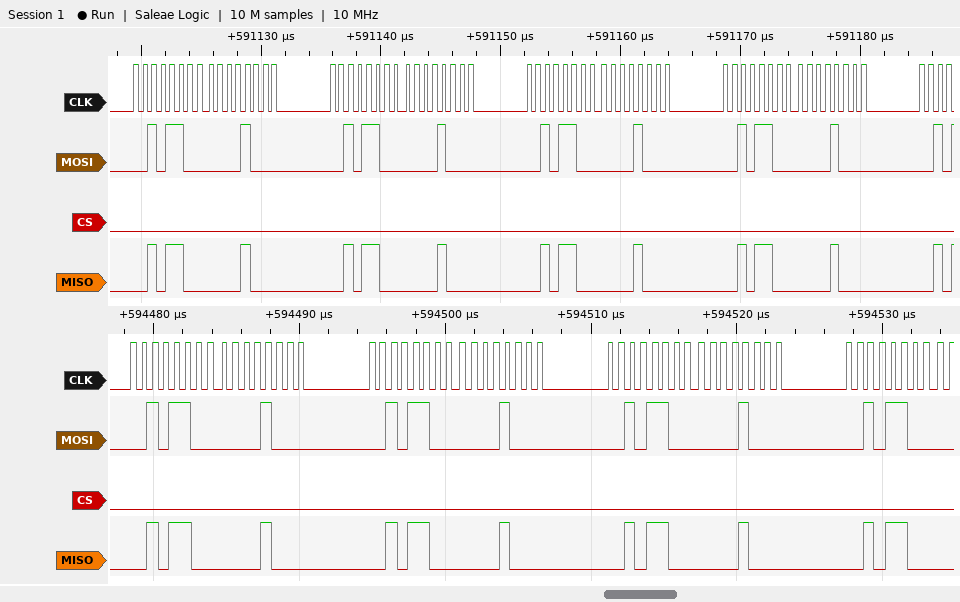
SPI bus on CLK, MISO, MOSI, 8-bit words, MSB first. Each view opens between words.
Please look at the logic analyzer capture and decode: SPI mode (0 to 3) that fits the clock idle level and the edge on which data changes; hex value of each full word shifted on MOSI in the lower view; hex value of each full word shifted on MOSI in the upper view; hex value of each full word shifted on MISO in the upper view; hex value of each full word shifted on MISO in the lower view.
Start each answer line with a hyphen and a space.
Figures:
- 0
- 2C, 08, 2C, 08, 2C, 08, 2C
- 2C, 08, 2C, 08, 2C, 08, 2C, 08
- 2C, 08, 2C, 08, 2C, 08, 2C, 08
- 2C, 08, 2C, 08, 2C, 08, 2C
